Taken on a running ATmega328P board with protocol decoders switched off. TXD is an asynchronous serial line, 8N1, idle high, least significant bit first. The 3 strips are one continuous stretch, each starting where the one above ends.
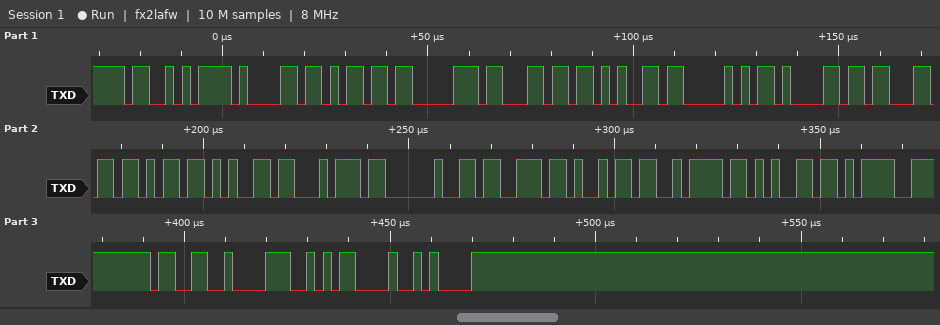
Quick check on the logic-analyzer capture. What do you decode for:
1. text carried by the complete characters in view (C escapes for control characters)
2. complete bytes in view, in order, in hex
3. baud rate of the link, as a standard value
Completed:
"SamplePacket size=38\r\n"
0x53 0x61 0x6D 0x70 0x6C 0x65 0x50 0x61 0x63 0x6B 0x65 0x74 0x20 0x73 0x69 0x7A 0x65 0x3D 0x33 0x38 0x0D 0x0A
500000 baud
